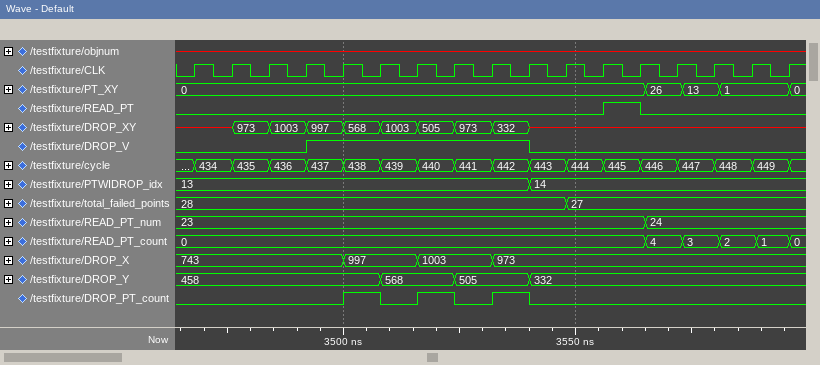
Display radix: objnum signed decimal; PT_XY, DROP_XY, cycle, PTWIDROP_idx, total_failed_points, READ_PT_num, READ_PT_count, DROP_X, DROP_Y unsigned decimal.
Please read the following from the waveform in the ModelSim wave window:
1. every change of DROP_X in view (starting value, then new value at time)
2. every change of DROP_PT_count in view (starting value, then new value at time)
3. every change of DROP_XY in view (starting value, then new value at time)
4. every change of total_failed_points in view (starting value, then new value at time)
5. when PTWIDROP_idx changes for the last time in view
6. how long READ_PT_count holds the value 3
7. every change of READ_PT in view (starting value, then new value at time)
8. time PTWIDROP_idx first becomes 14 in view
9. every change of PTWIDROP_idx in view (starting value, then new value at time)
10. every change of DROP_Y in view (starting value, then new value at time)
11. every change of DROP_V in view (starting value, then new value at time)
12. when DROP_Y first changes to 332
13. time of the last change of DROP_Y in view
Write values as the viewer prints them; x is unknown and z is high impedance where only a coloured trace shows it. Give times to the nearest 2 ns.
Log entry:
743, 997 at 3500 ns, 1003 at 3516 ns, 973 at 3532 ns
0, 1 at 3500 ns, 0 at 3508 ns, 1 at 3516 ns, 0 at 3524 ns, 1 at 3532 ns, 0 at 3540 ns
x, 973 at 3476 ns, 1003 at 3484 ns, 997 at 3492 ns, 568 at 3500 ns, 1003 at 3508 ns, 505 at 3516 ns, 973 at 3524 ns, 332 at 3532 ns, x at 3540 ns
28, 27 at 3548 ns
3540 ns
8 ns
0, 1 at 3556 ns, 0 at 3564 ns
3540 ns
13, 14 at 3540 ns
458, 568 at 3508 ns, 505 at 3524 ns, 332 at 3540 ns
0, 1 at 3492 ns, 0 at 3540 ns
3540 ns
3540 ns
